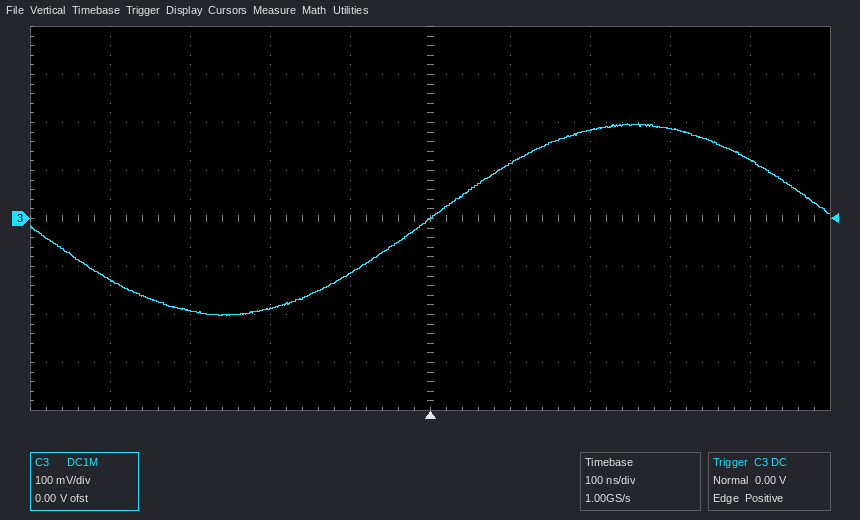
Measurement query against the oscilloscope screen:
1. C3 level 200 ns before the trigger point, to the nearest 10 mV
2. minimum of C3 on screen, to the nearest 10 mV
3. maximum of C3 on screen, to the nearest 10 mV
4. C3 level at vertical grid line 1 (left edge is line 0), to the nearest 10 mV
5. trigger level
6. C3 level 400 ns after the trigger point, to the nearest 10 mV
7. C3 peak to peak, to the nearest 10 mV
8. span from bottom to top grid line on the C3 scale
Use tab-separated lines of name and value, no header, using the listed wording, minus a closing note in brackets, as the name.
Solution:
C3 level 200 ns before the trigger point, to the nearest 10 mV	-190 mV
minimum of C3 on screen, to the nearest 10 mV	-200 mV
maximum of C3 on screen, to the nearest 10 mV	200 mV
C3 level at vertical grid line 1 (left edge is line 0), to the nearest 10 mV	-130 mV
trigger level	0.00 V
C3 level 400 ns after the trigger point, to the nearest 10 mV	120 mV
C3 peak to peak, to the nearest 10 mV	400 mV
span from bottom to top grid line on the C3 scale	800 mV
